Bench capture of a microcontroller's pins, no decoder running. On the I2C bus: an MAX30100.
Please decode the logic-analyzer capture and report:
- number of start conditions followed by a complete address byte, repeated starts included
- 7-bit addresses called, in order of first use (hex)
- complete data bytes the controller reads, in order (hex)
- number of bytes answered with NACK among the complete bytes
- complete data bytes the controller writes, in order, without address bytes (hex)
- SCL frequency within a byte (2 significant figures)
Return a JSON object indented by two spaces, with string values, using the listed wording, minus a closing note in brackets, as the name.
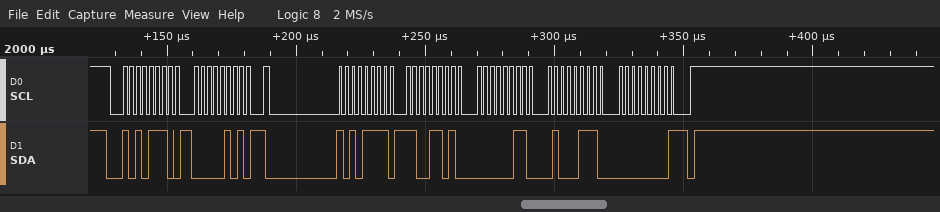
{
  "number of start conditions followed by a complete address byte, repeated starts included": "2",
  "7-bit addresses called, in order of first use": "0x57",
  "complete data bytes the controller reads, in order": "CD 03 47 00",
  "number of bytes answered with NACK among the complete bytes": "1",
  "complete data bytes the controller writes, in order, without address bytes": "05",
  "SCL frequency within a byte": "400 kHz"
}
